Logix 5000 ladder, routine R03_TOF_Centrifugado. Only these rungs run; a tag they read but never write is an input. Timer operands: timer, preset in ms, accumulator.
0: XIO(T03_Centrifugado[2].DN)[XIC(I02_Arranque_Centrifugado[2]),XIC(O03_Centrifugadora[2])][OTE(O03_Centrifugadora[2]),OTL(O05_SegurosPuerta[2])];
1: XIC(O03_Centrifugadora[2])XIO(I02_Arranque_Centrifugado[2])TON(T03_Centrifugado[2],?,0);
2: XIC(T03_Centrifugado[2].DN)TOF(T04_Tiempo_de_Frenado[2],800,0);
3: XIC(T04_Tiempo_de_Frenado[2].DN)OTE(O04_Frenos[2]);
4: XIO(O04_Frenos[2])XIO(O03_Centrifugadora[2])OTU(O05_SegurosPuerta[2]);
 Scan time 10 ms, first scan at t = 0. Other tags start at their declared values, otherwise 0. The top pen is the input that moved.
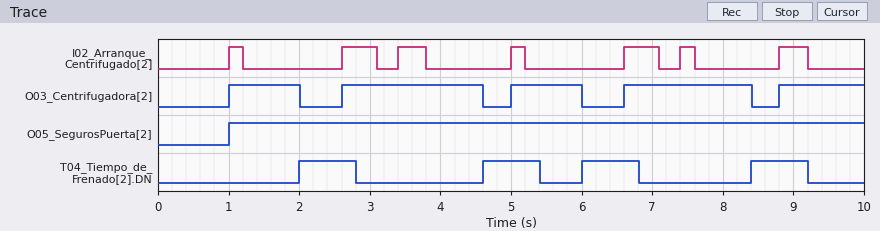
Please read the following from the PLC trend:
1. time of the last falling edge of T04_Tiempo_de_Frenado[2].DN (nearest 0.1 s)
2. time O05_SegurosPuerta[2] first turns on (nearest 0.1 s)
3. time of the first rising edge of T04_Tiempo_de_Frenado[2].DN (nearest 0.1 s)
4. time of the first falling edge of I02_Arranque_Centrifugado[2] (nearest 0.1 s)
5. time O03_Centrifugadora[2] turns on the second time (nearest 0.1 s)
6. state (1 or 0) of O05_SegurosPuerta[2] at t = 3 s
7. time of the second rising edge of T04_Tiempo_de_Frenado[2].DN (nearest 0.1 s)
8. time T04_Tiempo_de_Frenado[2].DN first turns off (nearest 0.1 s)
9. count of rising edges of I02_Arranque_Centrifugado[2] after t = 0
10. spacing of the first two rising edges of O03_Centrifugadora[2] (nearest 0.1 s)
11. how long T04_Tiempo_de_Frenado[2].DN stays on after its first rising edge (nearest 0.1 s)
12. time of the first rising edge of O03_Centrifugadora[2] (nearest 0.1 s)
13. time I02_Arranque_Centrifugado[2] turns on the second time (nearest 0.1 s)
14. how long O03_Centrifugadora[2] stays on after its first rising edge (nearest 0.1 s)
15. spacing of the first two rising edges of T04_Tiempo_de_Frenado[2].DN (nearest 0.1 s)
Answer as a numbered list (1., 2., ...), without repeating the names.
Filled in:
1. 9.2 s
2. 1.0 s
3. 2.0 s
4. 1.2 s
5. 2.6 s
6. 1
7. 4.6 s
8. 2.8 s
9. 7
10. 1.6 s
11. 0.8 s
12. 1.0 s
13. 2.6 s
14. 1.0 s
15. 2.6 s
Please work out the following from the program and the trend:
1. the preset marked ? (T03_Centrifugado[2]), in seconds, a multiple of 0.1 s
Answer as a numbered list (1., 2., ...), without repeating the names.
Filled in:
1. 0.8 s
